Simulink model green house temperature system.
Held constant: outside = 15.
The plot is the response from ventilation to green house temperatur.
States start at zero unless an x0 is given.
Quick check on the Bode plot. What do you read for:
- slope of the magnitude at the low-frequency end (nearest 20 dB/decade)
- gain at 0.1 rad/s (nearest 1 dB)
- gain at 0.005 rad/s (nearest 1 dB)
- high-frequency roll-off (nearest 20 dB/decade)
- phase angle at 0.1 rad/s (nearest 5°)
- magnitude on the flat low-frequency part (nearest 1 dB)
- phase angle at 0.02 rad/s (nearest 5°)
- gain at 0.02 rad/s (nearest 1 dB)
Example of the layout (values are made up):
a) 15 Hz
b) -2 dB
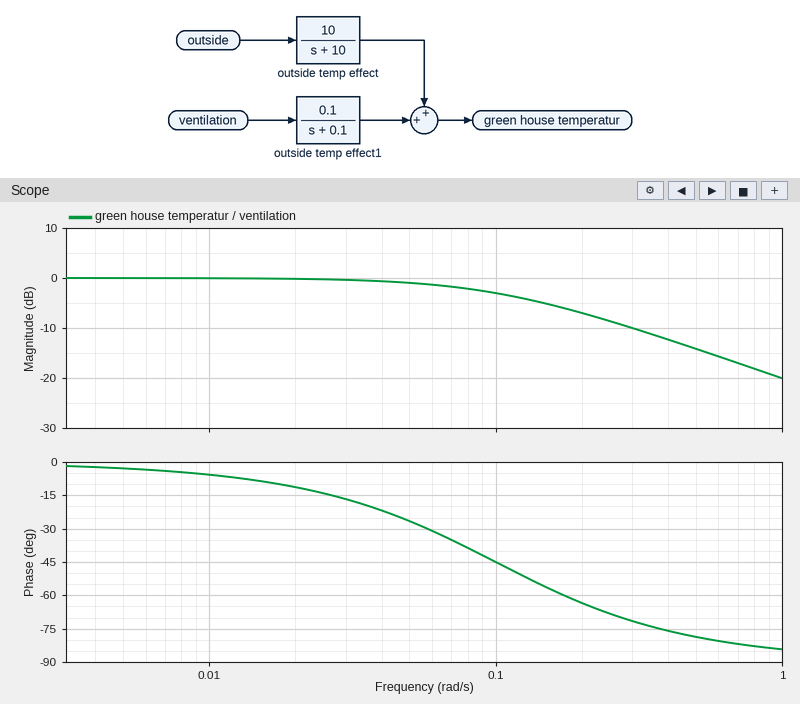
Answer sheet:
a) 0 dB/decade
b) -3 dB
c) 0 dB
d) -20 dB/decade
e) -45°
f) 0 dB
g) -10°
h) 0 dB
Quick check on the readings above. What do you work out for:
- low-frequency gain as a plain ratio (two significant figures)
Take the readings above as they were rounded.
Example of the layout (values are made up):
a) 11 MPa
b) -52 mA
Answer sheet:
a) 1.0
